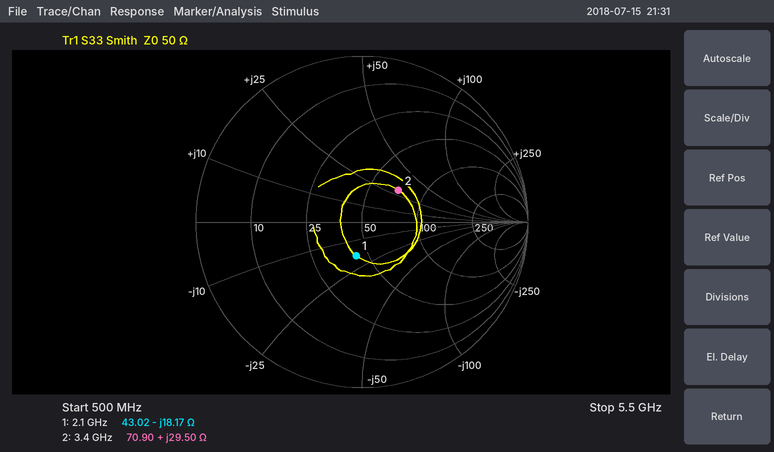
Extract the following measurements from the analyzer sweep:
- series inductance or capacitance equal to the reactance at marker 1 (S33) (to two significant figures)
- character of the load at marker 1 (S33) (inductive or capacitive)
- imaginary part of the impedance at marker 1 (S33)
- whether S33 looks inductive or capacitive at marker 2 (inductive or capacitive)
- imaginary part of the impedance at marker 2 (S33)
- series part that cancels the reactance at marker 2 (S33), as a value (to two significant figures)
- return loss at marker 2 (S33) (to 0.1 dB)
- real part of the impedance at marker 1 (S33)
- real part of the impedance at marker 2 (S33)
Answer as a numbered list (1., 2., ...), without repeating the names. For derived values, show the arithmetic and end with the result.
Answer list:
1. C = 1/(2π × 2.1 GHz × 18.17 Ω) ≈ 4.2 pF
2. capacitive
3. -18.17 Ω
4. inductive
5. +29.50 Ω
6. C = 1/(2π × 3.4 GHz × 29.5 Ω) ≈ 1.6 pF
7. 10.7 dB
8. 43.02 Ω
9. 70.90 Ω
